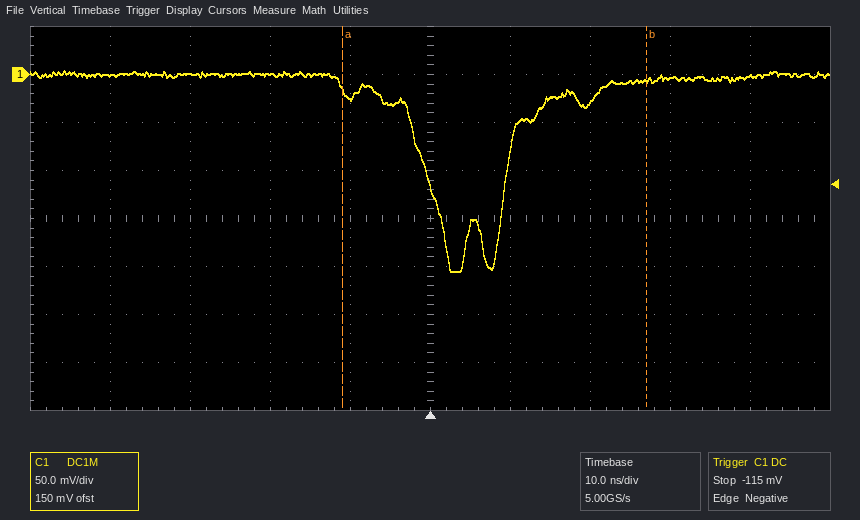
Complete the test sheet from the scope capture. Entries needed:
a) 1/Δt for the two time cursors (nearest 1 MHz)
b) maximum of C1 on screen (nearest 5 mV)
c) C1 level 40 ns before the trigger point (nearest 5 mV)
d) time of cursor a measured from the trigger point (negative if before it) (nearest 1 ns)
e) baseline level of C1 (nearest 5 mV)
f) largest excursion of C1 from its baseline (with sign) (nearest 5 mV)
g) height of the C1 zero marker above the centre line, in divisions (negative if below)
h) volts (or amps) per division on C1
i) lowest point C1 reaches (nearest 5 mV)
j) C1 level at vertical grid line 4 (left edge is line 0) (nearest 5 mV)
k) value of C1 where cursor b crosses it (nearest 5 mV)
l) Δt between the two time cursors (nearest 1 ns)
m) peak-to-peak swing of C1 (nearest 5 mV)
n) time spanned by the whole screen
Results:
26 MHz
5 mV
0 mV
-11 ns
0 mV
-205 mV
+3.0 div
50 mV
-205 mV
-25 mV
-5 mV
38 ns
210 mV
100 ns
